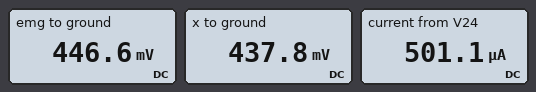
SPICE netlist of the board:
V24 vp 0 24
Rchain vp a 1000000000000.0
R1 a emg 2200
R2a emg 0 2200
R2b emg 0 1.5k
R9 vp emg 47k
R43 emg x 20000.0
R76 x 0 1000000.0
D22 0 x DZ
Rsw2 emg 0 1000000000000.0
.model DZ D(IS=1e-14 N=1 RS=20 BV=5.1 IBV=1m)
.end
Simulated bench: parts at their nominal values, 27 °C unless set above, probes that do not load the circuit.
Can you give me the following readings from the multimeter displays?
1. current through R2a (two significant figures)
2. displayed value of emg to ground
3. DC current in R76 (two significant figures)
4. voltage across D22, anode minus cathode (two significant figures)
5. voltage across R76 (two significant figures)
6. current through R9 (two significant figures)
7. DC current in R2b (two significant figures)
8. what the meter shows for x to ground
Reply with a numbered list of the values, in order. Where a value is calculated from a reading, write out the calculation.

1. (446.6 mV) / 2.2 kΩ = 200 µA
2. 446.6 mV
3. (437.8 mV) / 1 MΩ = 440 nA
4. 0 V - 437.8 mV = -440 mV
5. 437.8 mV = 440 mV
6. (24 V - 446.6 mV) / 47 kΩ = 500 µA
7. (446.6 mV) / 1.5 kΩ = 300 µA
8. 437.8 mV
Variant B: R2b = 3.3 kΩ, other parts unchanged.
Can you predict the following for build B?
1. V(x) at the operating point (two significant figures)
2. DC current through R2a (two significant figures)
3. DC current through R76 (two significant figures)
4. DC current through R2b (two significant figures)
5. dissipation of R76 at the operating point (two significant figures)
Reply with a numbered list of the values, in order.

1. 640 mV
2. 300 µA
3. 640 nA
4. 200 µA
5. 410 nW
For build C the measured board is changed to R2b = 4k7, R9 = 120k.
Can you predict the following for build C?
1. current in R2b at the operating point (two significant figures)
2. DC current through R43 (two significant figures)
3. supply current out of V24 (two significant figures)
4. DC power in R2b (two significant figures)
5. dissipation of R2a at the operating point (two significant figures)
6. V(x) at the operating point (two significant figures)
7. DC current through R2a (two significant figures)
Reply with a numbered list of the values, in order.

1. 63 µA
2. 290 nA
3. 200 µA
4. 19 µW
5. 40 µW
6. 290 mV
7. 130 µA
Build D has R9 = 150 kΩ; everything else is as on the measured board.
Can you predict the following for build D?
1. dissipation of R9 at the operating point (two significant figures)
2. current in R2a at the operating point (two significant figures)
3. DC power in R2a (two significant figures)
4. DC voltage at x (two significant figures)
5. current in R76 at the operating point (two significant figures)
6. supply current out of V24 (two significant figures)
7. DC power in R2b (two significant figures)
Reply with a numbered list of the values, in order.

1. 3.8 mW
2. 64 µA
3. 9.1 µW
4. 140 mV
5. 140 nA
6. 160 µA
7. 13 µW
